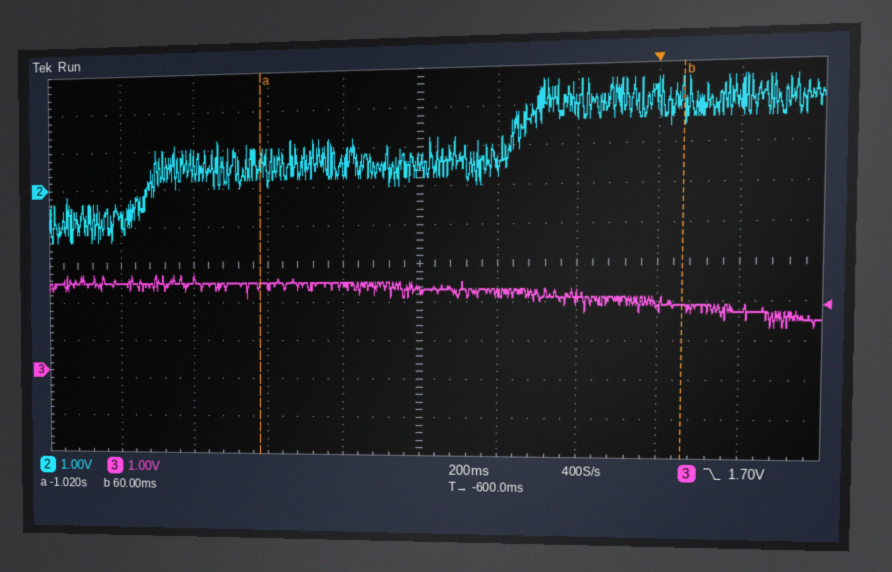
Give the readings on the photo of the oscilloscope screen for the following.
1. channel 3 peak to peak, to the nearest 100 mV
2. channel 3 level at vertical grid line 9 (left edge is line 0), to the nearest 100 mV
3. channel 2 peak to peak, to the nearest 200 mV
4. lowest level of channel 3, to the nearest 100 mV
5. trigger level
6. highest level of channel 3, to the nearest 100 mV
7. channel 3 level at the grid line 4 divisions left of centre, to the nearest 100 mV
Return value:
1.4 V
1.5 V
4.0 V
1.1 V
1.70 V
2.5 V
2.3 V
